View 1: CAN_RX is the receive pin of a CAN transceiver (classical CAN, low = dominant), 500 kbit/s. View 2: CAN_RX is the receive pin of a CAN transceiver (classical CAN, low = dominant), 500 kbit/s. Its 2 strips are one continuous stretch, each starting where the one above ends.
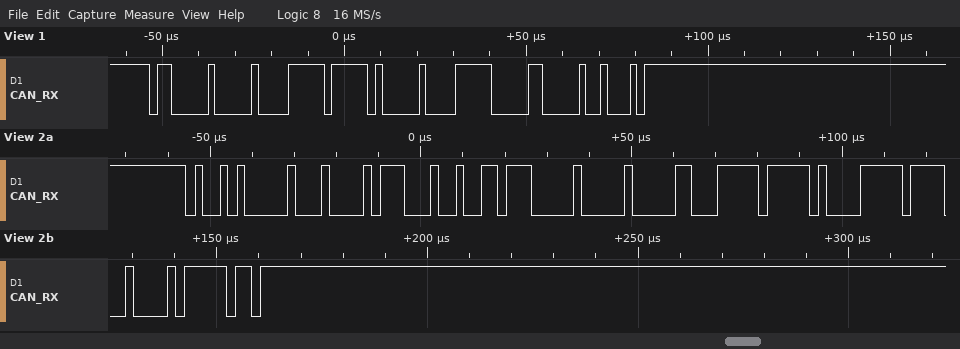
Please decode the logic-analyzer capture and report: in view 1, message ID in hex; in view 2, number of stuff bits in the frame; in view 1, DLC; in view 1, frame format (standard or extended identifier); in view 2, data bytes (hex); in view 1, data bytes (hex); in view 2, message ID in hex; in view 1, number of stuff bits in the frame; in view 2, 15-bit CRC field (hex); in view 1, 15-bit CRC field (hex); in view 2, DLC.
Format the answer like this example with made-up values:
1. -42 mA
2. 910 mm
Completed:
1. 0x600
2. 8
3. 3
4. standard
5. 5C 49 B8 00 08 FF E1 FF
6. FF 80 3E
7. 0x4A0
8. 8
9. 0x10BF
10. 0x0808
11. 8
